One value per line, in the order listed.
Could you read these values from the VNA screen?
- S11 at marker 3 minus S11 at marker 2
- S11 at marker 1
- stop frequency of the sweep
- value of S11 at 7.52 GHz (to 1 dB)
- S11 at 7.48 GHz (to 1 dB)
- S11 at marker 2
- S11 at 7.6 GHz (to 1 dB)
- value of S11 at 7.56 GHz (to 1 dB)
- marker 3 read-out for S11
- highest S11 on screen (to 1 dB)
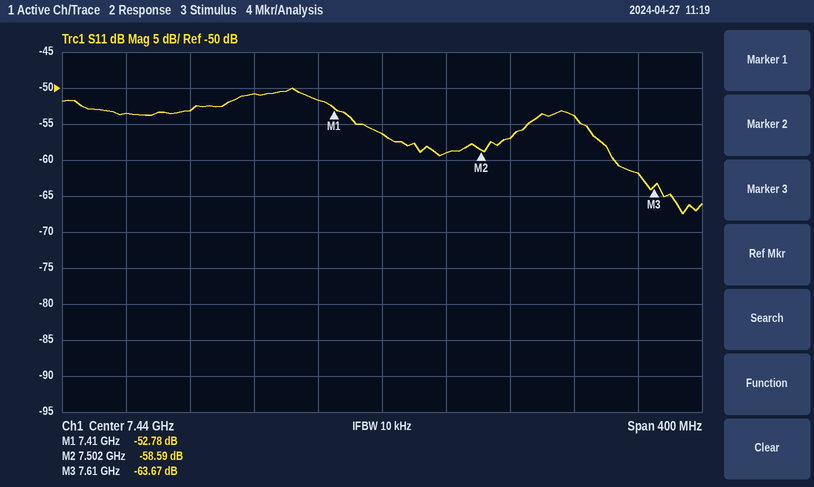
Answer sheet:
-5.08 dB
-52.78 dB
7.64 GHz
-57 dB
-59 dB
-58.59 dB
-62 dB
-54 dB
-63.67 dB
-50 dB
